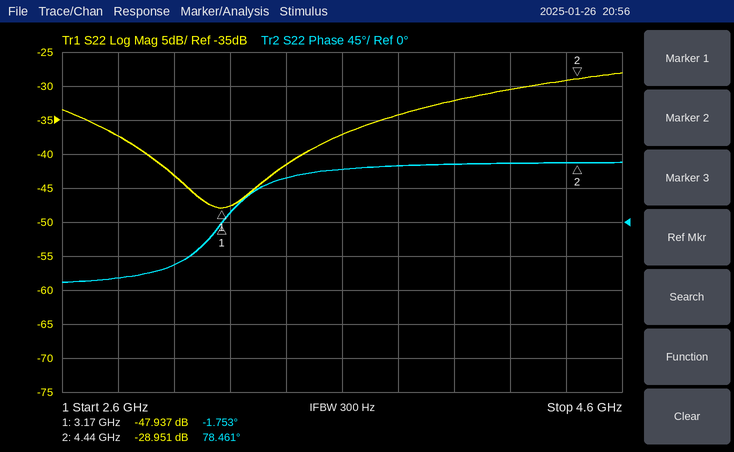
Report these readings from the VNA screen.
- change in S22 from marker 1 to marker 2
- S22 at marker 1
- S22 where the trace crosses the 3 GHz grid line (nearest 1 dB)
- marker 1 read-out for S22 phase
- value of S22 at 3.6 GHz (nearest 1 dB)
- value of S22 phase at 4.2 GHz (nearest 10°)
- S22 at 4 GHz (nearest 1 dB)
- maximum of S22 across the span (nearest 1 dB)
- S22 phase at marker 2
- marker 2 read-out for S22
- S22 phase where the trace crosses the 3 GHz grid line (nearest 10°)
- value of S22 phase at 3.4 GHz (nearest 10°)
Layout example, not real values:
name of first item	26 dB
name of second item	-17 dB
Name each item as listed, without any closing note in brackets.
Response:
change in S22 from marker 1 to marker 2	18.986 dB
S22 at marker 1	-47.937 dB
S22 where the trace crosses the 3 GHz grid line	-43 dB
marker 1 read-out for S22 phase	-1.753°
value of S22 at 3.6 GHz	-37 dB
value of S22 phase at 4.2 GHz	80°
S22 at 4 GHz	-32 dB
maximum of S22 across the span	-28 dB
S22 phase at marker 2	78.461°
marker 2 read-out for S22	-28.951 dB
S22 phase where the trace crosses the 3 GHz grid line	-60°
value of S22 phase at 3.4 GHz	60°
